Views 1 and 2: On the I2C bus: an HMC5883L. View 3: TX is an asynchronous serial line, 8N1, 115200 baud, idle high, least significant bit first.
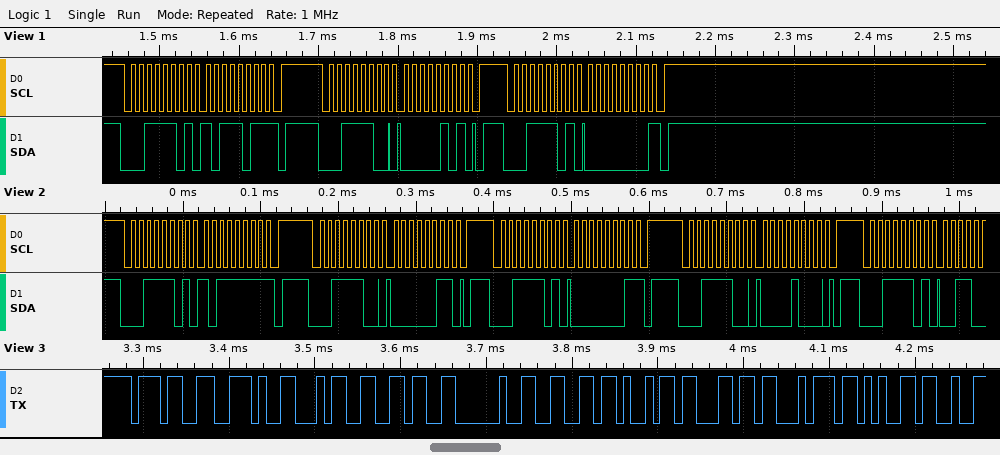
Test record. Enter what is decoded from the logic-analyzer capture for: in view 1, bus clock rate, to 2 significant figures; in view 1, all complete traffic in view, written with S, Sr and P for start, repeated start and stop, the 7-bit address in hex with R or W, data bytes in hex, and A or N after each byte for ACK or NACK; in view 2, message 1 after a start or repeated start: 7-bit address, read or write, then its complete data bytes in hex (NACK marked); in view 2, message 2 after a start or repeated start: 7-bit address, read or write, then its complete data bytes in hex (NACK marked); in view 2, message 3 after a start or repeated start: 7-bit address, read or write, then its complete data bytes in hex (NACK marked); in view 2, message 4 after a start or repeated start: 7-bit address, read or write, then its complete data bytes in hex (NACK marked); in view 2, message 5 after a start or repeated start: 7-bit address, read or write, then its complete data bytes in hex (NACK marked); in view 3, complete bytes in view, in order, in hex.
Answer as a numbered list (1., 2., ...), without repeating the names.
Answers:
1. 100 kHz
2. S 1ER A BB N P S 1EW A 05 A P S 1ER A 00 N P
3. 0x1E read: BF NACK
4. 0x1E write: 03
5. 0x1E read: 01 NACK
6. 0x1E write: 08
7. 0x1E read
8. 0x37 0x2E 0x34 0x36 0x20 0x66 0x69 0x6C 0x74 0x65
